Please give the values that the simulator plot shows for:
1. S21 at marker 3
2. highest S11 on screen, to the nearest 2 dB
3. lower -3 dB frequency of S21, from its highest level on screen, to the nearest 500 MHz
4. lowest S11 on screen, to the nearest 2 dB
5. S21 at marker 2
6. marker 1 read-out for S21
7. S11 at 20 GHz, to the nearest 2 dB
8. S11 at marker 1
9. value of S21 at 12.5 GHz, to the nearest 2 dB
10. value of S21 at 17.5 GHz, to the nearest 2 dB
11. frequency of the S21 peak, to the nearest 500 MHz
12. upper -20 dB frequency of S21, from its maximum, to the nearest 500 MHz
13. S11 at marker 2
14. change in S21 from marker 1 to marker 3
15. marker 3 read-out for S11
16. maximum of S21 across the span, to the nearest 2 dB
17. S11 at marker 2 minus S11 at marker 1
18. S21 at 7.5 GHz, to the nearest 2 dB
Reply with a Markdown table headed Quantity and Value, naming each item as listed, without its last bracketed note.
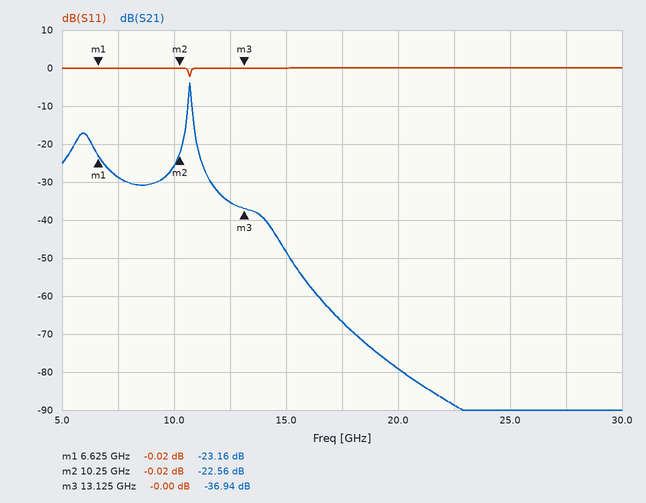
| Quantity | Value |
|---|---|
| S21 at marker 3 | -36.94 dB |
| highest S11 on screen, to the nearest 2 dB | 0 dB |
| lower -3 dB frequency of S21, from its highest level on screen, to the nearest 500 MHz | 10.5 GHz |
| lowest S11 on screen, to the nearest 2 dB | -2 dB |
| S21 at marker 2 | -22.56 dB |
| marker 1 read-out for S21 | -23.16 dB |
| S11 at 20 GHz, to the nearest 2 dB | 0 dB |
| S11 at marker 1 | -0.02 dB |
| value of S21 at 12.5 GHz, to the nearest 2 dB | -36 dB |
| value of S21 at 17.5 GHz, to the nearest 2 dB | -66 dB |
| frequency of the S21 peak, to the nearest 500 MHz | 10.5 GHz |
| upper -20 dB frequency of S21, from its maximum, to the nearest 500 MHz | 11.0 GHz |
| S11 at marker 2 | -0.02 dB |
| change in S21 from marker 1 to marker 3 | -13.78 dB |
| marker 3 read-out for S11 | -0.00 dB |
| maximum of S21 across the span, to the nearest 2 dB | -4 dB |
| S11 at marker 2 minus S11 at marker 1 | 0.00 dB |
| S21 at 7.5 GHz, to the nearest 2 dB | -28 dB |
